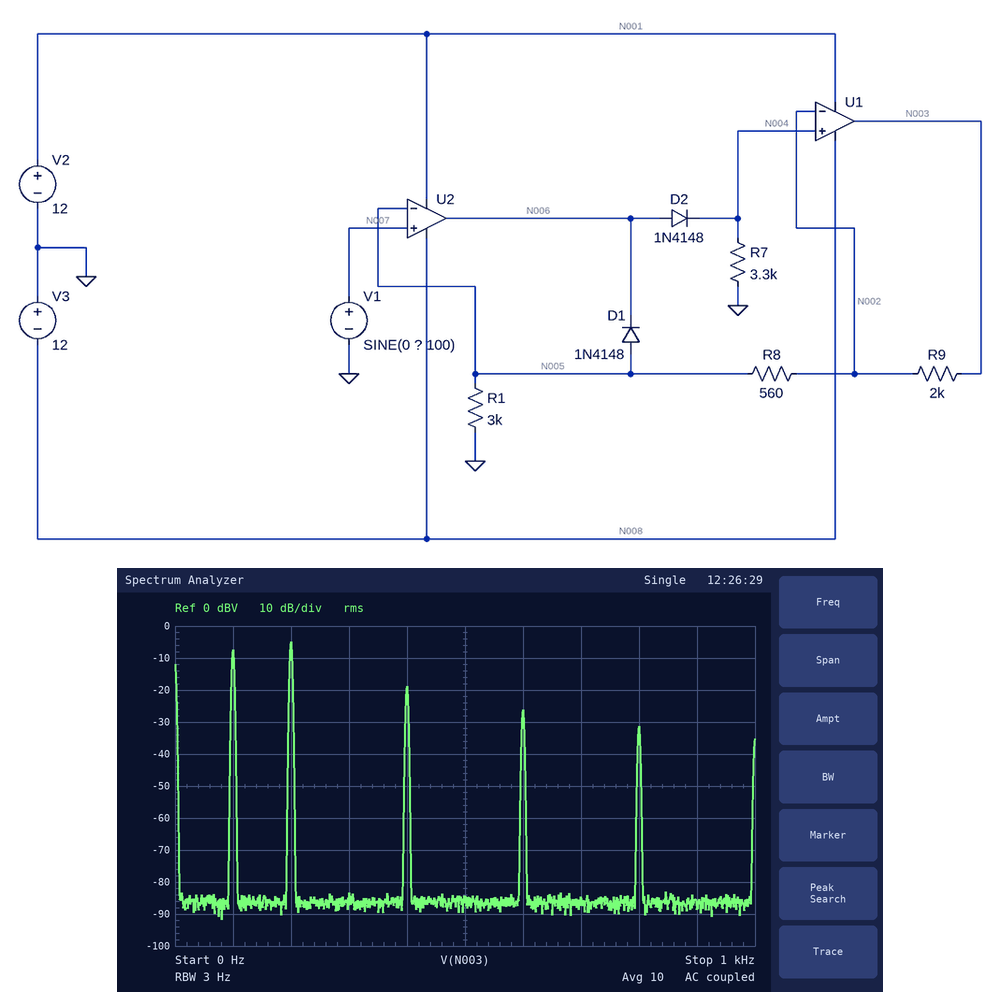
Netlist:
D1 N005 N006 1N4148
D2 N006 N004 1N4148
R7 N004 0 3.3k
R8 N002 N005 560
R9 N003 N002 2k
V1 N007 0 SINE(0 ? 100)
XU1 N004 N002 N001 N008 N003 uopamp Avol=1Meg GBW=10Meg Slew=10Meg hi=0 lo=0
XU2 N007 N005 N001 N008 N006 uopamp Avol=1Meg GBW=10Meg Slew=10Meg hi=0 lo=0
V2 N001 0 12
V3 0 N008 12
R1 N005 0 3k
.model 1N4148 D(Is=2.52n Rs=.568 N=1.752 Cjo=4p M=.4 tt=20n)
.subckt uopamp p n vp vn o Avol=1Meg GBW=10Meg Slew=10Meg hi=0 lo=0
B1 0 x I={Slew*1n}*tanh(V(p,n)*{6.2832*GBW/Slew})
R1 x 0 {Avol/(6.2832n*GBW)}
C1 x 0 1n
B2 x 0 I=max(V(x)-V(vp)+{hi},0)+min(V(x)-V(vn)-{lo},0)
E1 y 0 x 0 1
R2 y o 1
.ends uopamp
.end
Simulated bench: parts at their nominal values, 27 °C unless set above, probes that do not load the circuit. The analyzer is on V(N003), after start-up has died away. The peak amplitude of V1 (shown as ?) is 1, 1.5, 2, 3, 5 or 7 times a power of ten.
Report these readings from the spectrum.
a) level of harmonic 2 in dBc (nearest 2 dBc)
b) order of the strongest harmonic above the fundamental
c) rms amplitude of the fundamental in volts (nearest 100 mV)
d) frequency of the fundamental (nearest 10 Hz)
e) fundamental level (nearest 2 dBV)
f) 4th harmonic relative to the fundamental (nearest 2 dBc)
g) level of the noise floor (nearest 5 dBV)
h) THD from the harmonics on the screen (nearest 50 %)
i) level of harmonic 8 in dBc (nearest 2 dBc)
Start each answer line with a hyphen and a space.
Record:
- 2 dBc
- 2
- 400 mV
- 100 Hz
- -8 dBV
- -12 dBc
- -85 dBV
- 150 %
- -24 dBc
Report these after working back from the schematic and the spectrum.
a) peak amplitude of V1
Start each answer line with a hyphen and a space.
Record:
- 700 mV
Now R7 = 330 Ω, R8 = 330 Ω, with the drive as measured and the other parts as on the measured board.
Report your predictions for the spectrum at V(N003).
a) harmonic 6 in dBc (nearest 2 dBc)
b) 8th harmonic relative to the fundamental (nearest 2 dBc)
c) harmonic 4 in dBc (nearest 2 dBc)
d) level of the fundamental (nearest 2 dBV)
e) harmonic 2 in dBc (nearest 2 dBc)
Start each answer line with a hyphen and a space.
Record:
- -24 dBc
- -28 dBc
- -16 dBc
- 0 dBV
- -2 dBc
